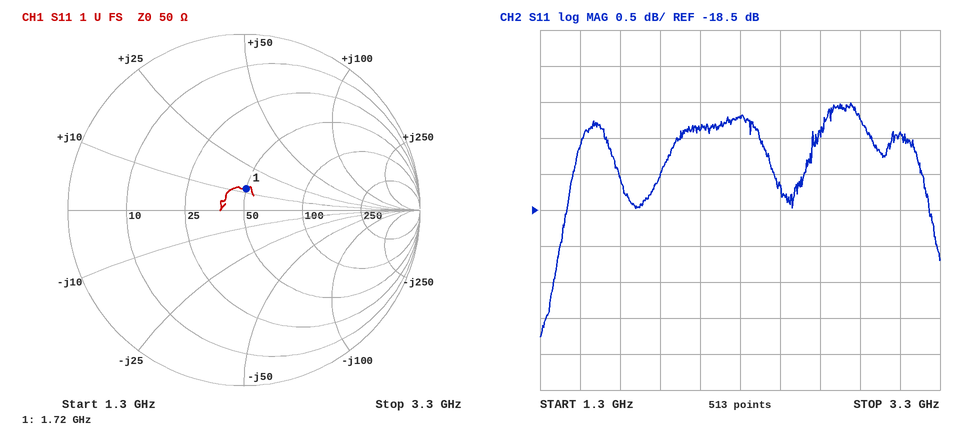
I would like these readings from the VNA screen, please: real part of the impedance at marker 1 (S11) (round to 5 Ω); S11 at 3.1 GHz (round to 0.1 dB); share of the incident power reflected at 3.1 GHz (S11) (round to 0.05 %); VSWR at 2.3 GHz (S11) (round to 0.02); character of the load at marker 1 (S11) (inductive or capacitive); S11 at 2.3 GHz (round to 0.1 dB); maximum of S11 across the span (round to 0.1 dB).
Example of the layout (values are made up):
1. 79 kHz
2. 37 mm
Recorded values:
1. 50 Ω
2. -17.4 dB
3. 1.80 %
4. 1.32
5. inductive
6. -17.2 dB
7. -17.0 dB
